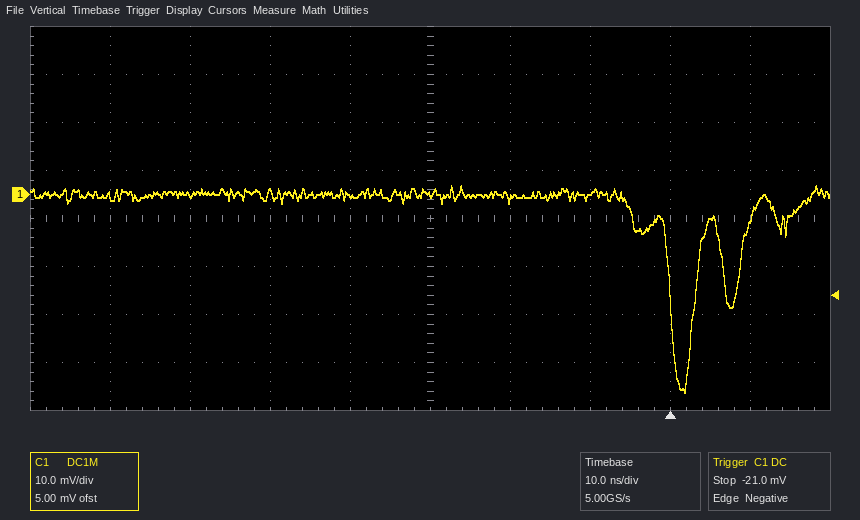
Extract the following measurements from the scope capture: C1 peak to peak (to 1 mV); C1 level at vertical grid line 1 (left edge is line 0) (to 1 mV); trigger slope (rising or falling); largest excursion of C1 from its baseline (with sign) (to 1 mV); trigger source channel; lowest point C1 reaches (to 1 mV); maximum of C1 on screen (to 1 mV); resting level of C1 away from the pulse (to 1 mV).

43 mV
0 mV
falling
-41 mV
C1
-41 mV
2 mV
0 mV
